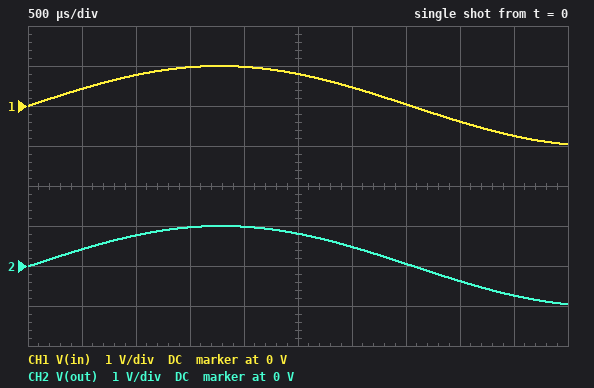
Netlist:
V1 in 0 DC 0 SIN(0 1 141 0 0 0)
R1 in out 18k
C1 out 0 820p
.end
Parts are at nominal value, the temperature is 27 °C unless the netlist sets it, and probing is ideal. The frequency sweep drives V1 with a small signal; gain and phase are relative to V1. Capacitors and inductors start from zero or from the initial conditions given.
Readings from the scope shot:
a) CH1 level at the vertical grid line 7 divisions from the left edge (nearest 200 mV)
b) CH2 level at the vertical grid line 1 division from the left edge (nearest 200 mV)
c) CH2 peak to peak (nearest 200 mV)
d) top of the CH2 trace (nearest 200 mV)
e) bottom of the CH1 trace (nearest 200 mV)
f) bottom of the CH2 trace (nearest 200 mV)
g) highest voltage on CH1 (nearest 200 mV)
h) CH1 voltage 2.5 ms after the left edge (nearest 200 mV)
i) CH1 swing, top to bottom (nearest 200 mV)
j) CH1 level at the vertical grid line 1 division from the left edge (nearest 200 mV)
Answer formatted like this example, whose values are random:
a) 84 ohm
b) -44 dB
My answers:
a) 0 V
b) 400 mV
c) 2.0 V
d) 1.0 V
e) -1.0 V
f) -1.0 V
g) 1.0 V
h) 800 mV
i) 2.0 V
j) 400 mV
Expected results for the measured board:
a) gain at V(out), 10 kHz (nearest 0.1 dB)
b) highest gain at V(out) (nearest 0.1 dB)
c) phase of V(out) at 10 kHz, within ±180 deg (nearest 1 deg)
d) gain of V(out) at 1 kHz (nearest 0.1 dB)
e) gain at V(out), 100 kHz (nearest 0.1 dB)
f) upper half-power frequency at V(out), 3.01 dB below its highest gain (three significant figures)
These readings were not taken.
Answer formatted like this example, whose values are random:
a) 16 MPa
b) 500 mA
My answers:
a) -2.7 dB
b) 0 dB
c) -43 deg
d) 0 dB
e) -19.4 dB
f) 10.8 kHz
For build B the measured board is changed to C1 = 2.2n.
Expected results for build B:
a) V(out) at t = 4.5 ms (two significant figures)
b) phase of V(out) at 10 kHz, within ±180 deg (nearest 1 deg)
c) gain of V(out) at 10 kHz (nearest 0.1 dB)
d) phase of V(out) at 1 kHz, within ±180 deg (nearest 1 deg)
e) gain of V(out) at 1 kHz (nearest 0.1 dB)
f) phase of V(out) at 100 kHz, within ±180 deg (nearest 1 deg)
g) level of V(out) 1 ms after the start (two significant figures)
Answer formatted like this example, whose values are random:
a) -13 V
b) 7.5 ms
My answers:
a) -720 mV
b) -68 deg
c) -8.6 dB
d) -14 deg
e) -0.3 dB
f) -88 deg
g) 750 mV
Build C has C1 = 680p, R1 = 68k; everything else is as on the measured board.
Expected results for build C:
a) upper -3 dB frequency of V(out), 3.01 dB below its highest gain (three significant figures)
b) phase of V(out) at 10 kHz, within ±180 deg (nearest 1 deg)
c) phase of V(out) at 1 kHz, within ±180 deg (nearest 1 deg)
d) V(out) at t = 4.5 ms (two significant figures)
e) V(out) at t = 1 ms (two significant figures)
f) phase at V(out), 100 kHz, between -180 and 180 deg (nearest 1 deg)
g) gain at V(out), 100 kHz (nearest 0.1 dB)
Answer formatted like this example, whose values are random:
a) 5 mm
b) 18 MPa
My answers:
a) 3.44 kHz
b) -71 deg
c) -16 deg
d) -720 mV
e) 750 mV
f) -88 deg
g) -29.3 dB
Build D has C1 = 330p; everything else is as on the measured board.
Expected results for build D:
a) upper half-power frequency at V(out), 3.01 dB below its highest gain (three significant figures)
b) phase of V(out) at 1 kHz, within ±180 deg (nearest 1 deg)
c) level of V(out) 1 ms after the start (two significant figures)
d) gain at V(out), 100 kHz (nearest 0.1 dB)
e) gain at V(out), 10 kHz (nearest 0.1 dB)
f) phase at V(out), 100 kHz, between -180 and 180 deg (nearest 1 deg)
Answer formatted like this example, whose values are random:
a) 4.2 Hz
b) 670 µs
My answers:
a) 26.8 kHz
b) -2 deg
c) 770 mV
d) -11.7 dB
e) -0.6 dB
f) -75 deg
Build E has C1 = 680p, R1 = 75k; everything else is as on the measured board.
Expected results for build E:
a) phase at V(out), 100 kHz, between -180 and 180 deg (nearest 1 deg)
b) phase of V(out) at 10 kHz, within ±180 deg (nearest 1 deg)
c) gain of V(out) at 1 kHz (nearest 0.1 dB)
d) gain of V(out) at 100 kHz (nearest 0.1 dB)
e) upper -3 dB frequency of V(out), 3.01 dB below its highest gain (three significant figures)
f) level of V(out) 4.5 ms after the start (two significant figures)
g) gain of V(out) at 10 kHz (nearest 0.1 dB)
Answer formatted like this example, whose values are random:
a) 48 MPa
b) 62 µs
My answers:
a) -88 deg
b) -73 deg
c) -0.4 dB
d) -30.1 dB
e) 3.12 kHz
f) -720 mV
g) -10.5 dB
